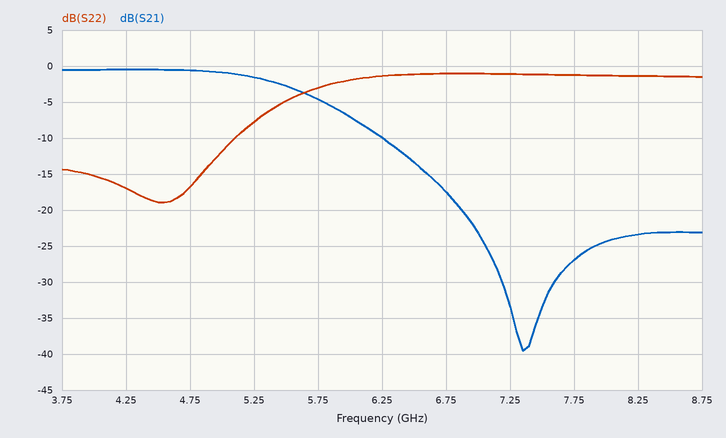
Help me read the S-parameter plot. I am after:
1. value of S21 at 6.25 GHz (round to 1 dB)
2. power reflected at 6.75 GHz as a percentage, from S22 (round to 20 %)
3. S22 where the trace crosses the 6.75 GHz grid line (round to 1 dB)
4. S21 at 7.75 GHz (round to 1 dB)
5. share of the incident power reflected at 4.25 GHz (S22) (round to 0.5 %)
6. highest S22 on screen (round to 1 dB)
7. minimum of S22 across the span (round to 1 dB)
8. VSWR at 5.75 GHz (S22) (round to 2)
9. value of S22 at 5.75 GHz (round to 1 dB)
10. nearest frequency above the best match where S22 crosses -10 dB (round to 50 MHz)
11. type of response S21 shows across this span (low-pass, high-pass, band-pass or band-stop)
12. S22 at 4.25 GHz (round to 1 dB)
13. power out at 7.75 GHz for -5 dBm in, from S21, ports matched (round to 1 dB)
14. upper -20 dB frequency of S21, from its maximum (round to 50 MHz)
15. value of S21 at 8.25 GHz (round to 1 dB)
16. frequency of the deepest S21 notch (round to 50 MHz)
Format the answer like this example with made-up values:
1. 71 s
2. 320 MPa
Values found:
1. -10 dB
2. 80 %
3. -1 dB
4. -27 dB
5. 2.0 %
6. -1 dB
7. -19 dB
8. 6
9. -3 dB
10. 5.10 GHz
11. low-pass
12. -17 dB
13. -32 dBm
14. 6.90 GHz
15. -23 dB
16. 7.35 GHz
